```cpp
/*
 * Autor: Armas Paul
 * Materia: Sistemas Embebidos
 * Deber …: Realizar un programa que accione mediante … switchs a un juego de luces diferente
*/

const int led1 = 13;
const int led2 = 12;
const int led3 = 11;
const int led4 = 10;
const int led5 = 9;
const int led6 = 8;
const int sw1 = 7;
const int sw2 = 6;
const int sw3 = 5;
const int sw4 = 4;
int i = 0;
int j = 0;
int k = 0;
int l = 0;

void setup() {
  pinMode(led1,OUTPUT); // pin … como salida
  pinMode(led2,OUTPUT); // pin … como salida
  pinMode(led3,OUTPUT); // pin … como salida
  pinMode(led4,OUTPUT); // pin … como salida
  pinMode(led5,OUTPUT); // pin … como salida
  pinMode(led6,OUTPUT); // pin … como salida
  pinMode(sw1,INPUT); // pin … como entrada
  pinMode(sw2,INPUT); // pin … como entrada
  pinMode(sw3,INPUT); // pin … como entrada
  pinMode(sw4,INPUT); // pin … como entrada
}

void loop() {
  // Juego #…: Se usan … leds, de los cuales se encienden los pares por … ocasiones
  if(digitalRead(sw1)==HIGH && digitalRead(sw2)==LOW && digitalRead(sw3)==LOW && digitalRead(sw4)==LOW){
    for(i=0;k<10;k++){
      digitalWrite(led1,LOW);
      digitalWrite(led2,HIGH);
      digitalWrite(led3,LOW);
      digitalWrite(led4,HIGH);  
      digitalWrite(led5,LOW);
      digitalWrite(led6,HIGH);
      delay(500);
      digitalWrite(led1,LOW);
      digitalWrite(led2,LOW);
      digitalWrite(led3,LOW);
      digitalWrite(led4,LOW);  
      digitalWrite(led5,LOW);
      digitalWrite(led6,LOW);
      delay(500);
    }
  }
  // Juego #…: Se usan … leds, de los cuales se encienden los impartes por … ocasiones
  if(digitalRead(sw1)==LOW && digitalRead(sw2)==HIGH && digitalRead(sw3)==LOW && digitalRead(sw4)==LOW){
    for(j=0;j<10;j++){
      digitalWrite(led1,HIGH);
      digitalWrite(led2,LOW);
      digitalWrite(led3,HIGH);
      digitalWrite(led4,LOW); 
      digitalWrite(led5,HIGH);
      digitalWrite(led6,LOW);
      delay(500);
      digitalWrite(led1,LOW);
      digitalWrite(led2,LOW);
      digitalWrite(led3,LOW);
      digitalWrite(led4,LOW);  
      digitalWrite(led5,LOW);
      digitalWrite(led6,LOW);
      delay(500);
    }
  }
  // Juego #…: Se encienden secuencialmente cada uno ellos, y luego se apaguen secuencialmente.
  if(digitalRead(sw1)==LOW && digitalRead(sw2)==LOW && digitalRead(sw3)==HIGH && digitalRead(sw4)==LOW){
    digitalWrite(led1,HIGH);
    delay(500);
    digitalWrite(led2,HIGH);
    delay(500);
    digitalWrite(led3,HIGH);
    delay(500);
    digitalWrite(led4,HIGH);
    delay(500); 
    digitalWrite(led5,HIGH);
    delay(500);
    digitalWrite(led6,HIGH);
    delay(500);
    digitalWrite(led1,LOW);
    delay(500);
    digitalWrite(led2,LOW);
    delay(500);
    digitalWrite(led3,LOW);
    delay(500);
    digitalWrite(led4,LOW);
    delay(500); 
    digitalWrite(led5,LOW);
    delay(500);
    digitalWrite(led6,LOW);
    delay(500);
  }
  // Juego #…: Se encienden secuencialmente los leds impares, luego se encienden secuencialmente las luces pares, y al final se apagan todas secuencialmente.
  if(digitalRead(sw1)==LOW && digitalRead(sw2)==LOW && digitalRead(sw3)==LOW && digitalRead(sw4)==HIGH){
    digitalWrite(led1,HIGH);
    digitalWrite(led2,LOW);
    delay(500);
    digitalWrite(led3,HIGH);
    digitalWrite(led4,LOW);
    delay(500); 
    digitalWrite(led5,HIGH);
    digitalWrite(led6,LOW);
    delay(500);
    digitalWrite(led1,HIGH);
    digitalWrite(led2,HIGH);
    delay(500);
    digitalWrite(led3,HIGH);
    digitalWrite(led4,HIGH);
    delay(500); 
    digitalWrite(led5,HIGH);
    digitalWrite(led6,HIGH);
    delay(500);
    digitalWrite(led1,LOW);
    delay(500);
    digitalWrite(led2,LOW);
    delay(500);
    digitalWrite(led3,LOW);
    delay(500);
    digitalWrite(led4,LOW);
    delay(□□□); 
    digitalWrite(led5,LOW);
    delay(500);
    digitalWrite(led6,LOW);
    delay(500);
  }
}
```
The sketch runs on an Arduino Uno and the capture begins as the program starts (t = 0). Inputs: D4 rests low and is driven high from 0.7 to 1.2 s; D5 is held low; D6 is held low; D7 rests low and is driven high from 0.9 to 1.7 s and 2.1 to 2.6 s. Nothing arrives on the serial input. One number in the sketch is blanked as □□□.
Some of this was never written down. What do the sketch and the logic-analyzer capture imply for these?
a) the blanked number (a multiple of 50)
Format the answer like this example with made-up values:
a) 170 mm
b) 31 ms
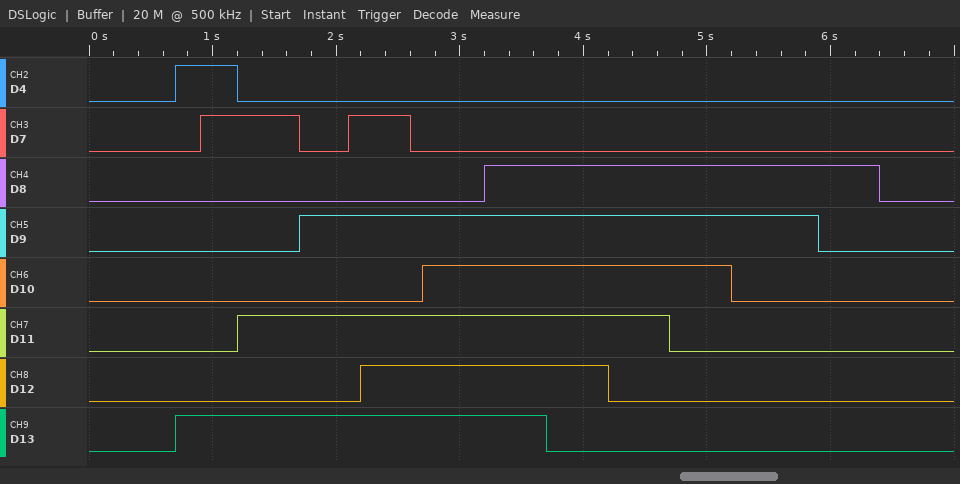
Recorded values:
a) 700
